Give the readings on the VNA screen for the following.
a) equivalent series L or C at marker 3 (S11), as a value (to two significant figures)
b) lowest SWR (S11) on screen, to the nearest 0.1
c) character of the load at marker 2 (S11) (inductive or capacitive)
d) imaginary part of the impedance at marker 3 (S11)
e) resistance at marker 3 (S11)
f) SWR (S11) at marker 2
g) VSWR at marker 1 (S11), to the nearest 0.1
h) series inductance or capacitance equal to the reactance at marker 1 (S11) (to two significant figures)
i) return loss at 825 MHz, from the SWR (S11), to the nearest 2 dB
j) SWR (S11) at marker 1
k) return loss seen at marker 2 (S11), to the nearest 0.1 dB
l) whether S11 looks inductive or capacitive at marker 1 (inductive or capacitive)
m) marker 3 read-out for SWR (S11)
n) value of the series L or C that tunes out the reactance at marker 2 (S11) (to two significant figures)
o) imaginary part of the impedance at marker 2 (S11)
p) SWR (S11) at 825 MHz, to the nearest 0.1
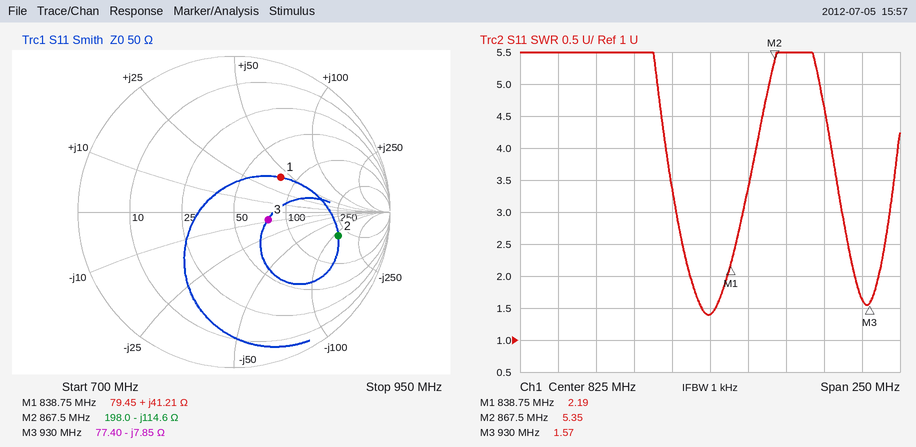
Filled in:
22 pF
1.4
capacitive
-7.85 Ω
77.40 Ω
5.35
2.2
7.8 nH
16 dB
2.19
3.3 dB
inductive
1.57
21 nH
-114.6 Ω
1.4
